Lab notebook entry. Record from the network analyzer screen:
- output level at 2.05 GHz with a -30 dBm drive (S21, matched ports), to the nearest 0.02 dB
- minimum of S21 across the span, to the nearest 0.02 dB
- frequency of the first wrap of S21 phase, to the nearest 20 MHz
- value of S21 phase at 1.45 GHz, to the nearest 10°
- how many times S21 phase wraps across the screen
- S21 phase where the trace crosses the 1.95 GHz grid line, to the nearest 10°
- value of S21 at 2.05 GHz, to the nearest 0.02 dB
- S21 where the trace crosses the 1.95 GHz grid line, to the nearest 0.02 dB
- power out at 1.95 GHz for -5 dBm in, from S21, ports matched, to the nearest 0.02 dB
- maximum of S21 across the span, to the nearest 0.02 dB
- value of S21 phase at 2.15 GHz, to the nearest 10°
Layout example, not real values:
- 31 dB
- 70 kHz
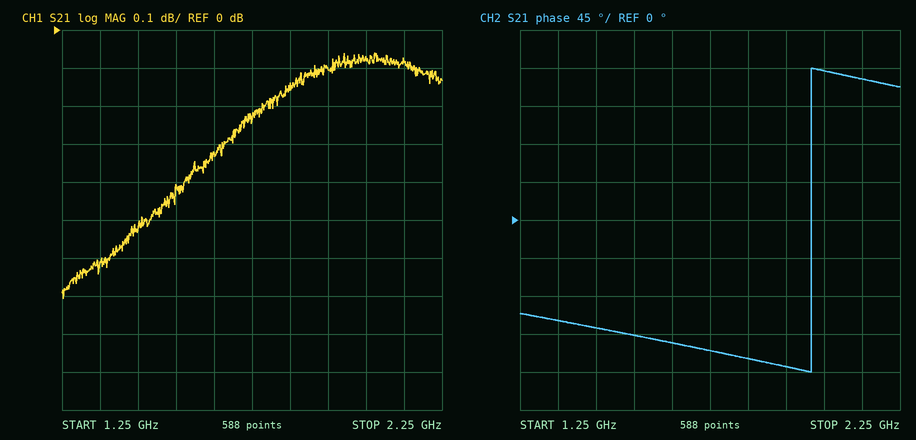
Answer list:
- -30.08 dBm
- -0.70 dB
- 2.02 GHz
- -130°
- 1
- -170°
- -0.08 dB
- -0.10 dB
- -5.10 dBm
- -0.06 dB
- 170°
